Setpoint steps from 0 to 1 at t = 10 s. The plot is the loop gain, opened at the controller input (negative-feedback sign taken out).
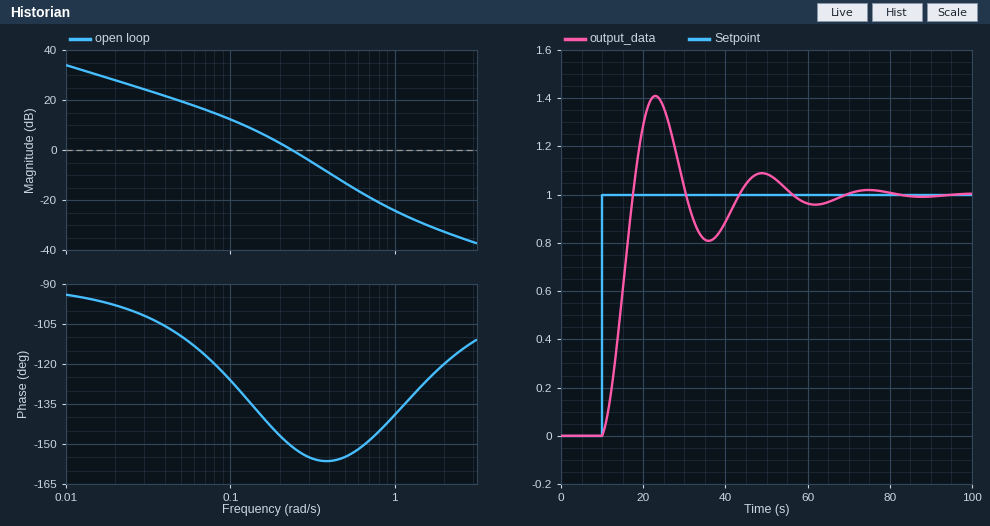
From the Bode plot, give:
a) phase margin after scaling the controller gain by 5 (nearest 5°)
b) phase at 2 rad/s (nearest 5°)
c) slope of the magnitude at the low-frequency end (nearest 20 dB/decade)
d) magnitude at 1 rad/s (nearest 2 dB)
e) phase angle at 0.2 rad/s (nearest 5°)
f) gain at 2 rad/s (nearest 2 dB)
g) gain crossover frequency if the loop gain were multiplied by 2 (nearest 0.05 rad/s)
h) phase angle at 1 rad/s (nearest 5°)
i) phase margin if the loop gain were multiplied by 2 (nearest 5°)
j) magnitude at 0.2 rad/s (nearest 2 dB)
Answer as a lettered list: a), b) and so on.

a) 25°
b) -120°
c) -20 dB/decade
d) -24 dB
e) -145°
f) -32 dB
g) 0.35 rad/s
h) -140°
i) 25°
j) 2 dB
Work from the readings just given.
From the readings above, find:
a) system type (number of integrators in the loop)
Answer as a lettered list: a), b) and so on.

a) 1
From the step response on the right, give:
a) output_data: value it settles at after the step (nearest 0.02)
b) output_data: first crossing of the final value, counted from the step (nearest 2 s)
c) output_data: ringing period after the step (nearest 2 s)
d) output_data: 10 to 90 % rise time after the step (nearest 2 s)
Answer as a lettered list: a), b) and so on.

a) 1.00
b) 8 s
c) 26 s
d) 6 s
